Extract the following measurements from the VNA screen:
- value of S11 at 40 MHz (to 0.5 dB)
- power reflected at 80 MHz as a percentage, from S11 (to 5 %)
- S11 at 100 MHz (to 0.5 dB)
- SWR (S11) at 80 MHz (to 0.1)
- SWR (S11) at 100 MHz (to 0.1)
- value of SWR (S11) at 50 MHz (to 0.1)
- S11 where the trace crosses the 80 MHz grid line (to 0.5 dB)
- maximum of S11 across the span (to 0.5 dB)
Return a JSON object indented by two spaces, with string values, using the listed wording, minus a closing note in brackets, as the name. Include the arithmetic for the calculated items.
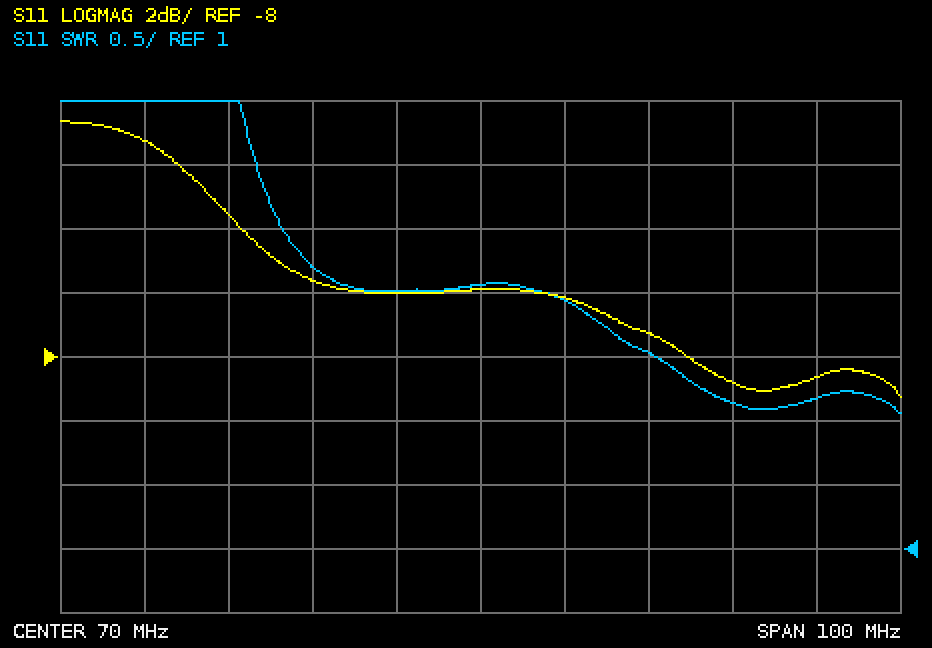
{
  "value of S11 at 40 MHz": "-3.5 dB",
  "power reflected at 80 MHz as a percentage, from S11": "10^(-6/10) ≈ 25 %",
  "S11 at 100 MHz": "-9.0 dB",
  "SWR (S11) at 80 MHz": "2.9",
  "SWR (S11) at 100 MHz": "2.1",
  "value of SWR (S11) at 50 MHz": "3.2",
  "S11 where the trace crosses the 80 MHz grid line": "-6.0 dB",
  "maximum of S11 across the span": "-0.5 dB"
}
